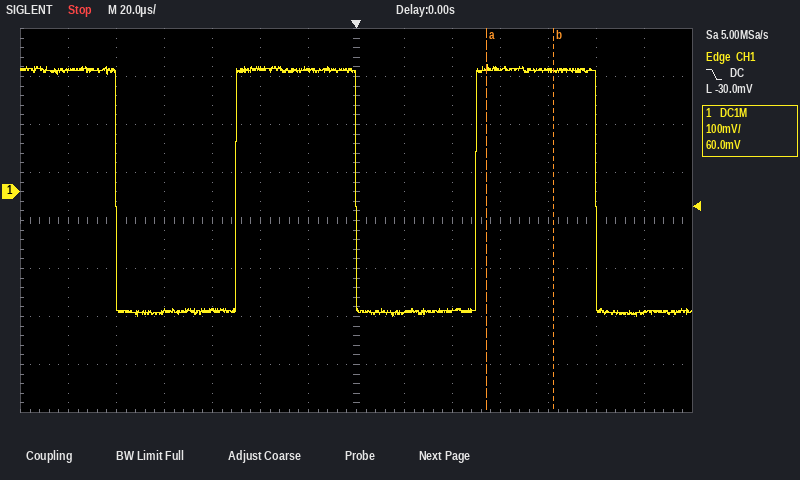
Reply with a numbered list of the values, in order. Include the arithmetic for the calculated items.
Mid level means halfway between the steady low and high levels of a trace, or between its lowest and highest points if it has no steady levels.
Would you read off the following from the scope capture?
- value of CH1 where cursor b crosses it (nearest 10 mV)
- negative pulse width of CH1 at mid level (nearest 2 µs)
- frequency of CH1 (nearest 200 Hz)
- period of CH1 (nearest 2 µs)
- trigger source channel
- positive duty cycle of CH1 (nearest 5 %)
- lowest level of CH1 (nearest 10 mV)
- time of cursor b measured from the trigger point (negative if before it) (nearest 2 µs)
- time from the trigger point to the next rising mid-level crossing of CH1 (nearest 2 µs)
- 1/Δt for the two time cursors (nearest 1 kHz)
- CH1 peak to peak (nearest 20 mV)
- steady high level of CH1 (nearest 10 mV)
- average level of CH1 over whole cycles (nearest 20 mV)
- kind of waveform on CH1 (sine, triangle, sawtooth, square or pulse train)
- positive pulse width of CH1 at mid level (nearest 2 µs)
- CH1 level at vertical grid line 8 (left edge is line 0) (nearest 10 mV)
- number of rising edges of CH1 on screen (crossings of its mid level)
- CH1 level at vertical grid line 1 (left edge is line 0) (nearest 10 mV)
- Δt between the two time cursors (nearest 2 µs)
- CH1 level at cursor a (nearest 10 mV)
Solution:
1. 250 mV
2. 50 µs
3. 1 / 100 µs ≈ 10.0 kHz
4. 100 µs
5. CH1
6. 50 µs / 100 µs ≈ 50 %
7. -260 mV
8. +82 µs
9. 50 µs
10. 1 / 28 µs ≈ 36 kHz
11. 520 mV
12. 250 mV
13. -260 mV + 0.5 × (250 mV − (-260 mV)) ≈ 0 mV
14. square
15. 50 µs
16. -250 mV
17. 2
18. 250 mV
19. 28 µs
20. 260 mV
